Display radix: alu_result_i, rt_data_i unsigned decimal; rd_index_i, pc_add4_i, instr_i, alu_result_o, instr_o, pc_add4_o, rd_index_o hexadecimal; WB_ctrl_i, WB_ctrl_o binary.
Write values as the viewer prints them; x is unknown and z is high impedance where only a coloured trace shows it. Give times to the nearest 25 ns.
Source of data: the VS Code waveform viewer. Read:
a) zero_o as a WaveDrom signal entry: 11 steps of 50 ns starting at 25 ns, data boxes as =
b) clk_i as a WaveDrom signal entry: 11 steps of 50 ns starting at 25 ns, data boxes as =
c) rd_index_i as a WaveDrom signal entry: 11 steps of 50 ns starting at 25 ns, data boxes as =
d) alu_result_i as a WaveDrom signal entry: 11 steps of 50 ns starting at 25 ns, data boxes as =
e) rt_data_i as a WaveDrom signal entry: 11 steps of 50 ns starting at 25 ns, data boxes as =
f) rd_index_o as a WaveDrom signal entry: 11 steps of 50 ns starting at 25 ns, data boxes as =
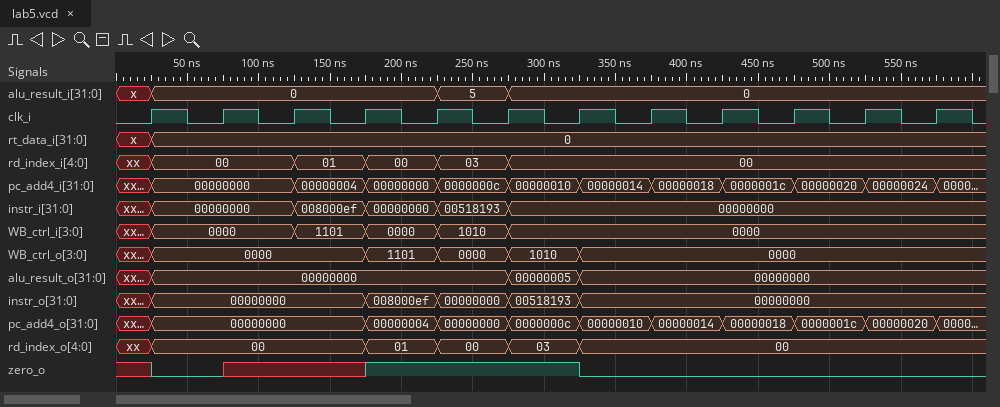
{name: 'zero_o', wave: '0x.1..0....'}
{name: 'clk_i', wave: 'p..........'}
{name: 'rd_index_i', wave: '=.====.....', data: '00 01 00 03 00'}
{name: 'alu_result_i', wave: '=...==.....', data: '0 5 0'}
{name: 'rt_data_i', wave: '=..........', data: '0'}
{name: 'rd_index_o', wave: '=..====....', data: '00 01 00 03 00'}
